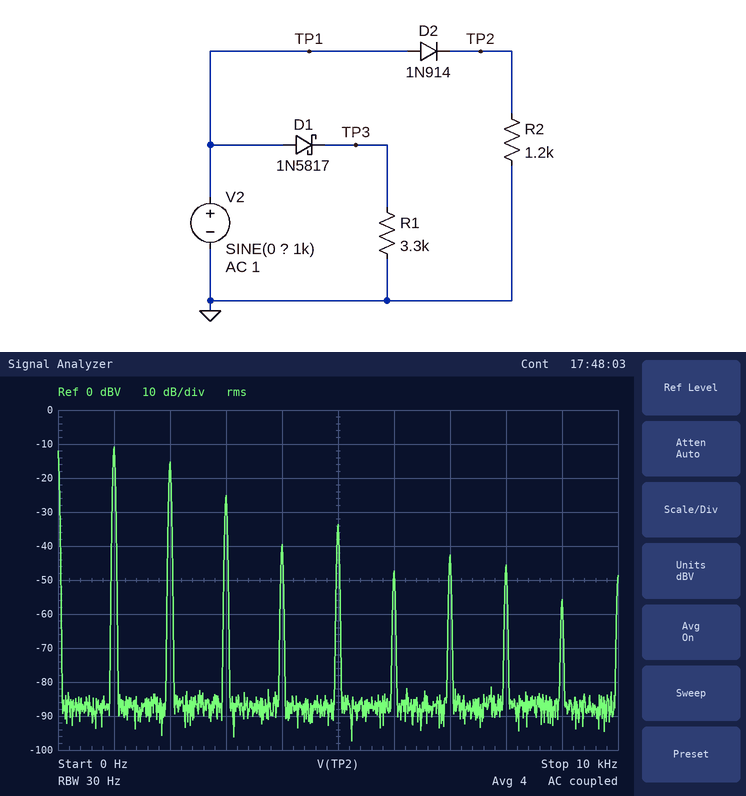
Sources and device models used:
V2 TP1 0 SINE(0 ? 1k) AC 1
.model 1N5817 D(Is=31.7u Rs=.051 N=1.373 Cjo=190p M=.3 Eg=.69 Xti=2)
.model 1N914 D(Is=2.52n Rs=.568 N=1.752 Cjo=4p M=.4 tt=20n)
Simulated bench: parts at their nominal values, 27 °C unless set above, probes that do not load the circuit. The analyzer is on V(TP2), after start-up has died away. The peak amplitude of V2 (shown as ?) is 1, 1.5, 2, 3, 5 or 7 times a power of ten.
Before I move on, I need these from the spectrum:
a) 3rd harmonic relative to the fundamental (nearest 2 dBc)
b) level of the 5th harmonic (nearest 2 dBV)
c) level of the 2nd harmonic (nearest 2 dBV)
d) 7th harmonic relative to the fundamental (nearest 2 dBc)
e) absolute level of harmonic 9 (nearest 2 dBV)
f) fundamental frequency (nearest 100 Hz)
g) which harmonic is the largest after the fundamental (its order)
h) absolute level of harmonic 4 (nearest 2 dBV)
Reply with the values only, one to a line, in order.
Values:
-14 dBc
-34 dBV
-16 dBV
-32 dBc
-56 dBV
1.0 kHz
2
-40 dBV
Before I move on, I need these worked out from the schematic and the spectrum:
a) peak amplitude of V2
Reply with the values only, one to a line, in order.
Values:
1.5 V
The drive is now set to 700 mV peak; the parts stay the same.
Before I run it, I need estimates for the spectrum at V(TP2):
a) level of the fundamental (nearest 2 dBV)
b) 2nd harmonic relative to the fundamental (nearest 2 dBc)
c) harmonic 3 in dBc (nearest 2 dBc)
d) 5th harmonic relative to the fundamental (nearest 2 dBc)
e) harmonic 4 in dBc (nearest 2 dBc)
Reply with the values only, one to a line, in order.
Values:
-26 dBV
-2 dBc
-8 dBc
-42 dBc
-16 dBc
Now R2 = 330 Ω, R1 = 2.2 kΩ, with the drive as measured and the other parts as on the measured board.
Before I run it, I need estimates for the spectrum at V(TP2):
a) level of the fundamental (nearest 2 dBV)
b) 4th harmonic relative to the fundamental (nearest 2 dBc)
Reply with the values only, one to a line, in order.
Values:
-12 dBV
-34 dBc
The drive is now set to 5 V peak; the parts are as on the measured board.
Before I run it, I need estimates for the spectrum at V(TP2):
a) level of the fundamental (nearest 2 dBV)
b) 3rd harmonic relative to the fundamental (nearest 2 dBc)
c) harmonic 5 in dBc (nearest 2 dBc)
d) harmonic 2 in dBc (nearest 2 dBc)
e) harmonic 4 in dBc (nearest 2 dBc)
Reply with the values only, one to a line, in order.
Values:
4 dBV
-26 dBc
-30 dBc
-6 dBc
-22 dBc
